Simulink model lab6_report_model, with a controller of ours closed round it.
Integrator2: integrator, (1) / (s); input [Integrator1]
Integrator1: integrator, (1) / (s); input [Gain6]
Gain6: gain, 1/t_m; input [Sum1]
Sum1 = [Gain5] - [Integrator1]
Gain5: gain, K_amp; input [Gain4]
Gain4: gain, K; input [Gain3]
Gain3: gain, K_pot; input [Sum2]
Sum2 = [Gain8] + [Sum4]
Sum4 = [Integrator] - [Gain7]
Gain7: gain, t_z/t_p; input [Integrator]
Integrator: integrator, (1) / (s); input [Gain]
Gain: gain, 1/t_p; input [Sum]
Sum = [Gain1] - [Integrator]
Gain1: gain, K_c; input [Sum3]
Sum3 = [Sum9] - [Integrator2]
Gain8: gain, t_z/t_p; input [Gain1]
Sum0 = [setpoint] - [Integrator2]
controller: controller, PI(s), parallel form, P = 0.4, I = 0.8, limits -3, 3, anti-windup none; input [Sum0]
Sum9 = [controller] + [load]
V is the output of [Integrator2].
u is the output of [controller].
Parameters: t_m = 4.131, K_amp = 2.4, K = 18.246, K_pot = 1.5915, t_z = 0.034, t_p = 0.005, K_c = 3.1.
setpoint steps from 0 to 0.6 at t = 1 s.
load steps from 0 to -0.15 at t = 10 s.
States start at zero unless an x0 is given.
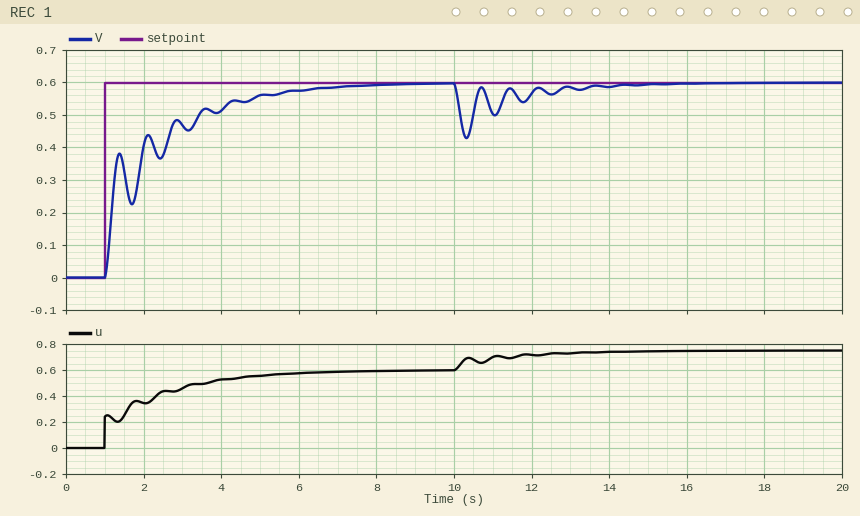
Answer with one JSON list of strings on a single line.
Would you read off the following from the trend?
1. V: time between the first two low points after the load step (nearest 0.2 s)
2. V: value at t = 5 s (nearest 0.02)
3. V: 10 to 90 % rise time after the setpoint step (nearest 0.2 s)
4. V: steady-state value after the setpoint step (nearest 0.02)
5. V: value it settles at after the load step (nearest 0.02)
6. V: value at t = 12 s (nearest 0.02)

["0.8 s", "0.56", "3.2 s", "0.60", "0.60", "0.56"]
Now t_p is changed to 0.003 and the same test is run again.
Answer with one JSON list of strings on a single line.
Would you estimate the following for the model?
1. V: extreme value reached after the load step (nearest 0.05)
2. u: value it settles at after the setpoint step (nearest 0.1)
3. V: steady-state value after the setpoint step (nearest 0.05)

["0.45", "0.6", "0.60"]
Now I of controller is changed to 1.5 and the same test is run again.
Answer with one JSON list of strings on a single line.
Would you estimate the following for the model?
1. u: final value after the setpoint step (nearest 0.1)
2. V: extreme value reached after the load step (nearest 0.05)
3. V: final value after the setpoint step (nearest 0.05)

["0.6", "0.45", "0.60"]
